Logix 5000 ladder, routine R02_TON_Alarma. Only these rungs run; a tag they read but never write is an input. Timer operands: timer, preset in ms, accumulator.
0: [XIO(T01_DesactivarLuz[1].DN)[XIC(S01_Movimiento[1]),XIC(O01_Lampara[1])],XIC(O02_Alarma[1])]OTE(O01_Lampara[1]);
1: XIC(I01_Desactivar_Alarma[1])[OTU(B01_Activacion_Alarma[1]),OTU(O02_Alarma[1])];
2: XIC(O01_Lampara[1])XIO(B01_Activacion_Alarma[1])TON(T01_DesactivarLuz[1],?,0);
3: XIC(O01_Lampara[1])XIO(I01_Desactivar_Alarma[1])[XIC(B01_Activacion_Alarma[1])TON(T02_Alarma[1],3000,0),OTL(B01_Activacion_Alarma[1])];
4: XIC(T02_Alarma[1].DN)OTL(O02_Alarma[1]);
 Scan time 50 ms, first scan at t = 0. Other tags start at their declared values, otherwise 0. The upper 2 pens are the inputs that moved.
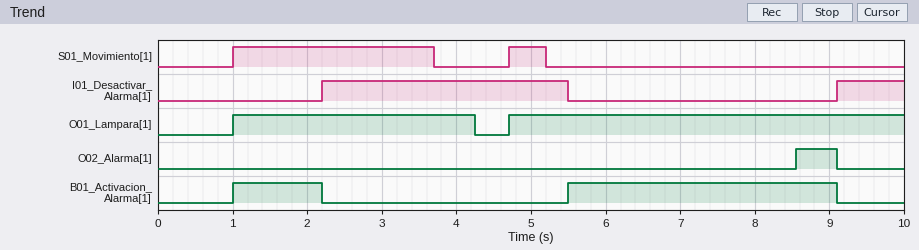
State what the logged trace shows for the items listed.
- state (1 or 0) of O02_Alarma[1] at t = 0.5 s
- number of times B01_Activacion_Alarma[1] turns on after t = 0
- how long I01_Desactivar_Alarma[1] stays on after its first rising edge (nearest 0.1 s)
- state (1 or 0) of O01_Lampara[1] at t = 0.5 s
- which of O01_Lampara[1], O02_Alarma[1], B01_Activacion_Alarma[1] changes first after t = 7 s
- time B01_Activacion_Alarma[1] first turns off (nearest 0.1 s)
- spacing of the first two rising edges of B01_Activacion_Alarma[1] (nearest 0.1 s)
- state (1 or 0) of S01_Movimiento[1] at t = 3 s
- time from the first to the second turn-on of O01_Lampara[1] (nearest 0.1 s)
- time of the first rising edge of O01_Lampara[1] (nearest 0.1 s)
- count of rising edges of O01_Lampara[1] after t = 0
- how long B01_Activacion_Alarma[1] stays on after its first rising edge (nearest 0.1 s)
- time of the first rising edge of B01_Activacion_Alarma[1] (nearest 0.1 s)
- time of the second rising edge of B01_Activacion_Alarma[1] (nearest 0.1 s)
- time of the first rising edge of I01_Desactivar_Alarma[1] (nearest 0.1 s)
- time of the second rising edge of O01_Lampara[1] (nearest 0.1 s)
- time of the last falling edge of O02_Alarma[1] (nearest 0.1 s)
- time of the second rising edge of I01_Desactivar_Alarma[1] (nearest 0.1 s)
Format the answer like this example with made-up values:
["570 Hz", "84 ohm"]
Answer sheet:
["0", "2", "3.3 s", "0", "O02_Alarma[1]", "2.2 s", "4.5 s", "1", "3.7 s", "1.0 s", "2", "1.2 s", "1.0 s", "5.5 s", "2.2 s", "4.7 s", "9.1 s", "9.1 s"]
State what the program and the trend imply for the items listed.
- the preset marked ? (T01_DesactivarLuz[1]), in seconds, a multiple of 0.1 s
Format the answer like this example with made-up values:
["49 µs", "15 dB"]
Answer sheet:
["2.0 s"]
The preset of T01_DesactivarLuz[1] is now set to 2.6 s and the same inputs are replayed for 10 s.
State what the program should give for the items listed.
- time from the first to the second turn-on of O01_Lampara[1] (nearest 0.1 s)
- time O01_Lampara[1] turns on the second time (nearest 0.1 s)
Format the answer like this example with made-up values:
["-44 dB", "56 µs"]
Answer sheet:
["3.9 s", "4.9 s"]
